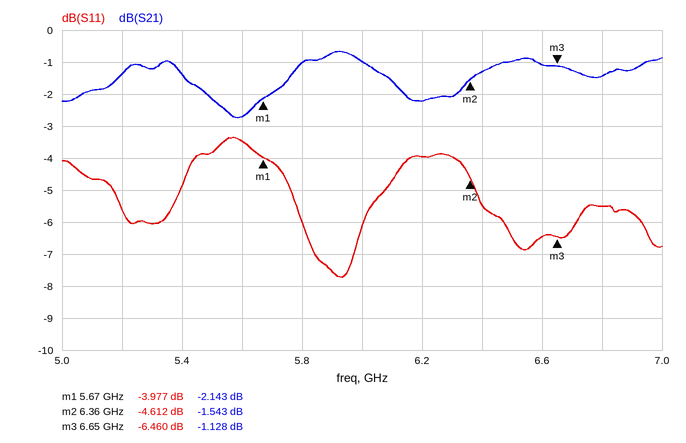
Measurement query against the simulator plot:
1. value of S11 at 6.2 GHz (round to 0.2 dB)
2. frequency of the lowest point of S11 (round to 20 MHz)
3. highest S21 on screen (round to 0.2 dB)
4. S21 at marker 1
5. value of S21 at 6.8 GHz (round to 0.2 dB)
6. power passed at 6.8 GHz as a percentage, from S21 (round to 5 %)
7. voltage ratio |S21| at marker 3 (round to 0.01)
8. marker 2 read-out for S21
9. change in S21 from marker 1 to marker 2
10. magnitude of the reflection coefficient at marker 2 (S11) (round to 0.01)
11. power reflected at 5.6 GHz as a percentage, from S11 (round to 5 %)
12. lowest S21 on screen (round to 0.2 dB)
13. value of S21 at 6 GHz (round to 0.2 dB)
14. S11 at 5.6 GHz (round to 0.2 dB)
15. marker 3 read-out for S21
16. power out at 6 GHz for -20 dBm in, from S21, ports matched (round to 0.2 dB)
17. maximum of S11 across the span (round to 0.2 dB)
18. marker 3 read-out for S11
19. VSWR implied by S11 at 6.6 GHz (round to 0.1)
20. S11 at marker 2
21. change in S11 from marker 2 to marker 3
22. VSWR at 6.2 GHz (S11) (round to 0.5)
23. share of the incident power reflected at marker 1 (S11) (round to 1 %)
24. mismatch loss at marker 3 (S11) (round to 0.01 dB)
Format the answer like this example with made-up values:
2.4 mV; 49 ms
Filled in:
-4.0 dB; 5.94 GHz; -0.6 dB; -2.143 dB; -1.4 dB; 70 %; 0.88; -1.543 dB; 0.600 dB; 0.59; 45 %; -2.8 dB; -1.0 dB; -3.4 dB; -1.128 dB; -21.0 dBm; -3.4 dB; -6.460 dB; 2.8; -4.612 dB; -1.848 dB; 4.5; 40 %; 1.11 dB
